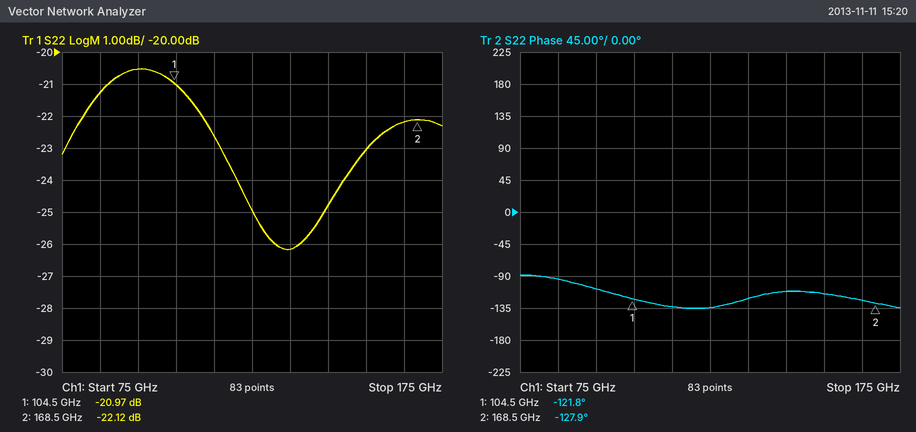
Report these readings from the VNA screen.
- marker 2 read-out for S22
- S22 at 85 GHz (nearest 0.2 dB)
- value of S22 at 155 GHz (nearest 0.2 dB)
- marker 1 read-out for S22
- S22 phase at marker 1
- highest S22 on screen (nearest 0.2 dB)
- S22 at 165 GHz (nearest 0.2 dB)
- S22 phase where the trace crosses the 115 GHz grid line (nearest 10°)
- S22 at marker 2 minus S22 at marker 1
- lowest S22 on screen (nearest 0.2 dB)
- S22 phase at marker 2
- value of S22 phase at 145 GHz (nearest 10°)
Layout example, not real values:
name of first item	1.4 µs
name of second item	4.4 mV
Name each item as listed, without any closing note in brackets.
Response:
marker 2 read-out for S22	-22.12 dB
S22 at 85 GHz	-21.2 dB
value of S22 at 155 GHz	-23.0 dB
marker 1 read-out for S22	-20.97 dB
S22 phase at marker 1	-121.8°
highest S22 on screen	-20.6 dB
S22 at 165 GHz	-22.2 dB
S22 phase where the trace crosses the 115 GHz grid line	-130°
S22 at marker 2 minus S22 at marker 1	-1.15 dB
lowest S22 on screen	-26.2 dB
S22 phase at marker 2	-127.9°
value of S22 phase at 145 GHz	-110°
